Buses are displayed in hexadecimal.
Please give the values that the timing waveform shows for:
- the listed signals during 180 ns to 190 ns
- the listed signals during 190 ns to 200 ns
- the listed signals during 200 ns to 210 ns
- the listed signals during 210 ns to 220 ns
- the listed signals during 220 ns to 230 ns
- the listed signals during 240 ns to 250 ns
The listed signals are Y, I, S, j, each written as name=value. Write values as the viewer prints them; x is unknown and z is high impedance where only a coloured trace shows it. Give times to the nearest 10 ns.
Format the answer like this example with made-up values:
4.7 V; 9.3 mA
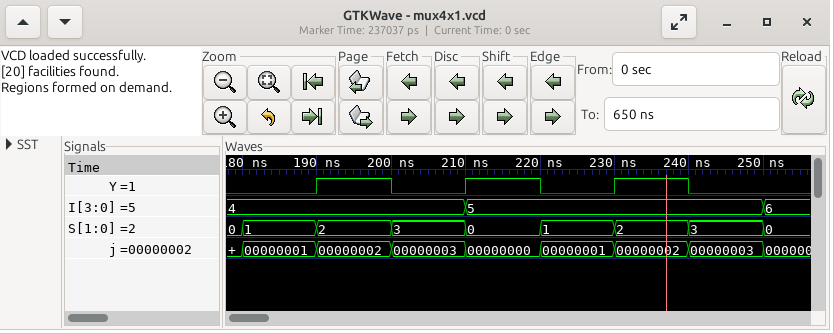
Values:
Y=0, I=4, S=1, j=00000001; Y=1, I=4, S=2, j=00000002; Y=0, I=4, S=3, j=00000003; Y=1, I=5, S=0, j=00000000; Y=0, I=5, S=1, j=00000001; Y=0, I=5, S=3, j=00000003
